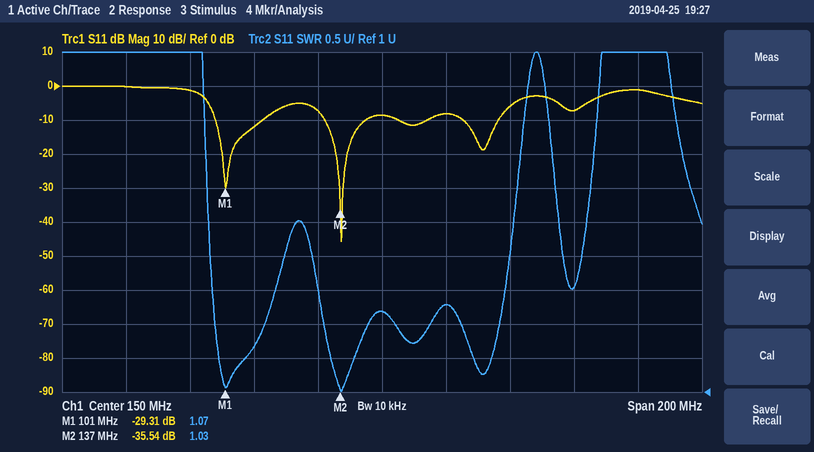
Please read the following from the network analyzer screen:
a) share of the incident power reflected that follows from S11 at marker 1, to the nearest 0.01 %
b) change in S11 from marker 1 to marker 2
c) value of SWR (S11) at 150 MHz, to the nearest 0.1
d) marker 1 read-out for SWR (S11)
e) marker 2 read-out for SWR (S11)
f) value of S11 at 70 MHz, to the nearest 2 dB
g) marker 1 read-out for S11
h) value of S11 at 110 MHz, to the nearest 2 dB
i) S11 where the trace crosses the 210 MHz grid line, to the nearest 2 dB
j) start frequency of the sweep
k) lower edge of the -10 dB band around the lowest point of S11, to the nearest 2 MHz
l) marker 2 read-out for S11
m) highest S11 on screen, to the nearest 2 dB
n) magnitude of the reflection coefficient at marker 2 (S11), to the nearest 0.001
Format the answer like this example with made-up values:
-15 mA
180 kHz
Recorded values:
0.12 %
-6.23 dB
2.2
1.07
1.03
0 dB
-29.31 dB
-12 dB
-8 dB
50 MHz
132 MHz
-35.54 dB
0 dB
0.017
